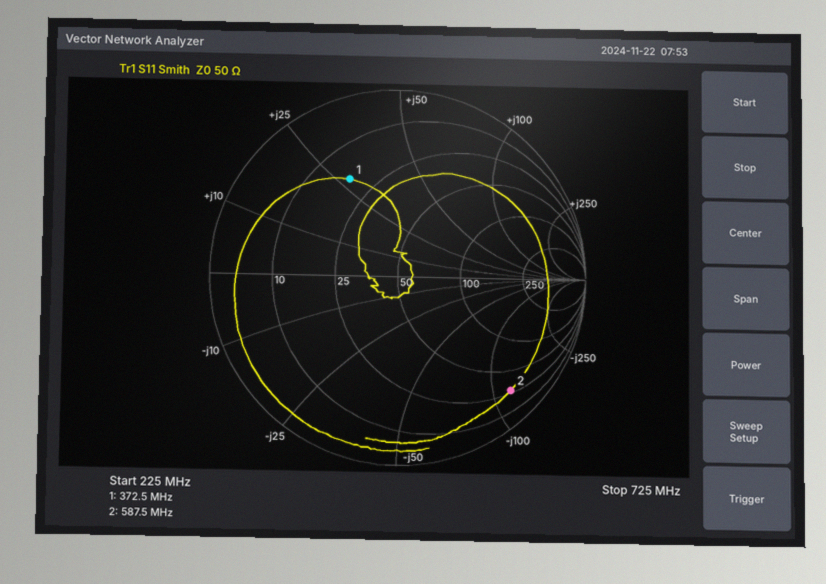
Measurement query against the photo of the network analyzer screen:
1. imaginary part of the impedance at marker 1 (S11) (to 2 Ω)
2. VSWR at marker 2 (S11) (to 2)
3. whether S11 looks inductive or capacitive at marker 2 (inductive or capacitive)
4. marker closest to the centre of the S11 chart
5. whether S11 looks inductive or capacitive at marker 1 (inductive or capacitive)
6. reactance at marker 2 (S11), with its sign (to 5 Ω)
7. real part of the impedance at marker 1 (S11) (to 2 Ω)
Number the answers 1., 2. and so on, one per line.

1. +28 Ω
2. 12
3. capacitive
4. marker 1
5. inductive
6. -115 Ω
7. 18 Ω
